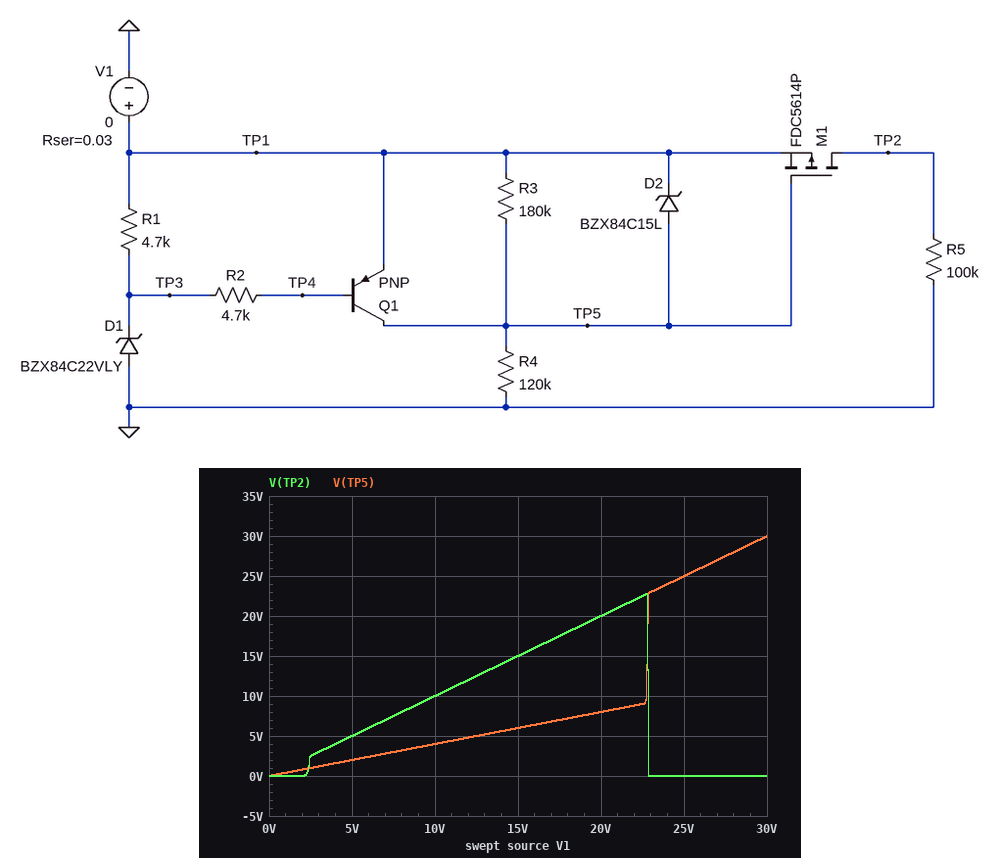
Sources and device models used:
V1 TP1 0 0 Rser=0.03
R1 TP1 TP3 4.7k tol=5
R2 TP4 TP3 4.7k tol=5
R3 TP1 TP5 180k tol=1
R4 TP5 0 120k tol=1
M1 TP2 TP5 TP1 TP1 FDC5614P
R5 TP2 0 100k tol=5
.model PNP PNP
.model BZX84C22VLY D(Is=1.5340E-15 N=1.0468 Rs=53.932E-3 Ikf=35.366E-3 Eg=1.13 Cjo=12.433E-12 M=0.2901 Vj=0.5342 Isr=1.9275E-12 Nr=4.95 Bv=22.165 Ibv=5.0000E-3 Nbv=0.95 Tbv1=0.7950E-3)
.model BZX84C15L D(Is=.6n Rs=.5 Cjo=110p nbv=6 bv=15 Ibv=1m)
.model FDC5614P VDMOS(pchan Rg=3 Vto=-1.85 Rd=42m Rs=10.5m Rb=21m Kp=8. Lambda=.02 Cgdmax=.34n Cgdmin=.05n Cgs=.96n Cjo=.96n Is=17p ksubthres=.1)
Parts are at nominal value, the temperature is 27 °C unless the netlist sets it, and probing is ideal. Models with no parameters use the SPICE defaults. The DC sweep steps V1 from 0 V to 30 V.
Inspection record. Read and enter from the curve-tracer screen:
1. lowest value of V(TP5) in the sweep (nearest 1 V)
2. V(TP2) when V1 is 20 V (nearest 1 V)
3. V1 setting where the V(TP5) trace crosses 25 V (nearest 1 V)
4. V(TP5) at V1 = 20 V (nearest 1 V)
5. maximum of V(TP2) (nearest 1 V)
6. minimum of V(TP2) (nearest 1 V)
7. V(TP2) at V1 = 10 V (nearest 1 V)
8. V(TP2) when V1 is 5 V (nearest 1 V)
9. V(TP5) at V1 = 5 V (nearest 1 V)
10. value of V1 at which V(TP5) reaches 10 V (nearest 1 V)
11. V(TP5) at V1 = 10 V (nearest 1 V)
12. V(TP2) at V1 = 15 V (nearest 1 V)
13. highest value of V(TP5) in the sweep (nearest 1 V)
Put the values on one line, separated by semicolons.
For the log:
0 V; 20 V; 25 V; 8 V; 23 V; 0 V; 10 V; 5 V; 2 V; 23 V; 4 V; 15 V; 30 V
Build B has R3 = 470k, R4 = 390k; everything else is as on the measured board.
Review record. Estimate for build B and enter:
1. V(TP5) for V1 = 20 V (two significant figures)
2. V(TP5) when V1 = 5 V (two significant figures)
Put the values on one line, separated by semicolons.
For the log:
9.1 V; 2.3 V
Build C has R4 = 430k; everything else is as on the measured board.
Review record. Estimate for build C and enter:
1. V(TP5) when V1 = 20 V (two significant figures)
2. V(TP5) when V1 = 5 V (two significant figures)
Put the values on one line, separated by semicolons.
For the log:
14 V; 3.5 V
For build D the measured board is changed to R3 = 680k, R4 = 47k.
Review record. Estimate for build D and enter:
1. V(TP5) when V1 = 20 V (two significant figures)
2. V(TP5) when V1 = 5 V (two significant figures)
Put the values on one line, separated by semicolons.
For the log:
5.4 V; 320 mV
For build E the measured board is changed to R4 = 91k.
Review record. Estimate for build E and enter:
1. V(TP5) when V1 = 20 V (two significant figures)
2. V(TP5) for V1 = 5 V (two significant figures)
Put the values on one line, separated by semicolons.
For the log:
6.7 V; 1.7 V
